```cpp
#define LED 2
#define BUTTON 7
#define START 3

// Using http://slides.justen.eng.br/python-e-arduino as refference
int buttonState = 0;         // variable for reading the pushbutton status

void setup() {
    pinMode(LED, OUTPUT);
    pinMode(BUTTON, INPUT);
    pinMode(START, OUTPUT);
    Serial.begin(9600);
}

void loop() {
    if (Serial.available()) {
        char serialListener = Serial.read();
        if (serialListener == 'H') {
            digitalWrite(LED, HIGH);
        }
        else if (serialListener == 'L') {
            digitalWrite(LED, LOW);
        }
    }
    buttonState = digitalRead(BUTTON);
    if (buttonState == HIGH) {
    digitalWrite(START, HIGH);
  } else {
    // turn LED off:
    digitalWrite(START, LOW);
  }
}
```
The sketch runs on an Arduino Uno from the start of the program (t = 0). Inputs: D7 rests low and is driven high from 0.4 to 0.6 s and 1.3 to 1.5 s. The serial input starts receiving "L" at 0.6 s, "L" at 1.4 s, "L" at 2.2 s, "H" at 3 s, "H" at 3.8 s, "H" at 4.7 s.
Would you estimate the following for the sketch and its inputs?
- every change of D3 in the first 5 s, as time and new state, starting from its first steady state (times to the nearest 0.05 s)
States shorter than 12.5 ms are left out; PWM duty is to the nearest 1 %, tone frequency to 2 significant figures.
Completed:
0 s low; 0.4 s high; 0.6 s low; 1.3 s high; 1.5 s low
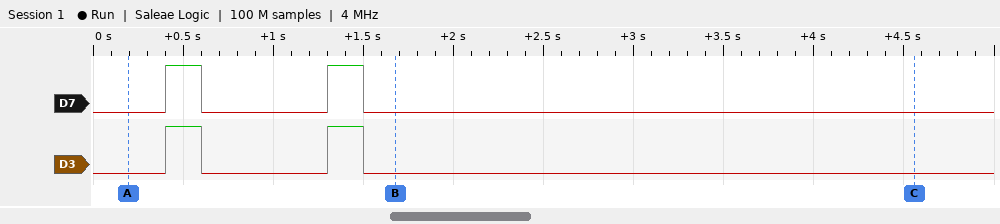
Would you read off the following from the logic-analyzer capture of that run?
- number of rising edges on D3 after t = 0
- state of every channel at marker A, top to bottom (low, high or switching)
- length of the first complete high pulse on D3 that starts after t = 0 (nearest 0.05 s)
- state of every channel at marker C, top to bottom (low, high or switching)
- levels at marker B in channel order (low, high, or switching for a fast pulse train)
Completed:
2
D7 low, D3 low
0.20 s
D7 low, D3 low
D7 low, D3 low
